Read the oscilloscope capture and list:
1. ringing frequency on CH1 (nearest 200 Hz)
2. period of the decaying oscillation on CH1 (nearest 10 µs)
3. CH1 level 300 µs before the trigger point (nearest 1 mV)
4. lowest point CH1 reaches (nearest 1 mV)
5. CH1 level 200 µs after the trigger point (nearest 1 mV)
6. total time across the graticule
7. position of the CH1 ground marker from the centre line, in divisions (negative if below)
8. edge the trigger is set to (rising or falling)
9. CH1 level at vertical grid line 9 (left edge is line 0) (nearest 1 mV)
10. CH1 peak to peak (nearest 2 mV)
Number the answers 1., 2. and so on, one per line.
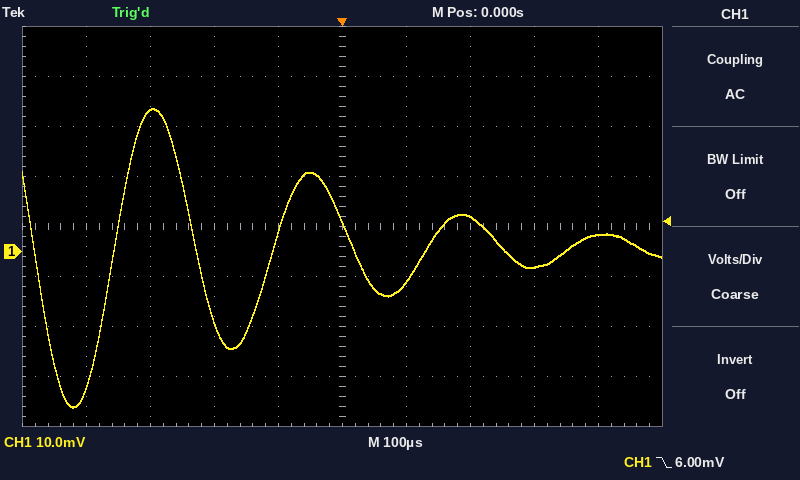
1. 4.2 kHz
2. 240 µs
3. 28 mV
4. -31 mV
5. 7 mV
6. 1 ms
7. -0.5 div
8. falling
9. 3 mV
10. 60 mV
